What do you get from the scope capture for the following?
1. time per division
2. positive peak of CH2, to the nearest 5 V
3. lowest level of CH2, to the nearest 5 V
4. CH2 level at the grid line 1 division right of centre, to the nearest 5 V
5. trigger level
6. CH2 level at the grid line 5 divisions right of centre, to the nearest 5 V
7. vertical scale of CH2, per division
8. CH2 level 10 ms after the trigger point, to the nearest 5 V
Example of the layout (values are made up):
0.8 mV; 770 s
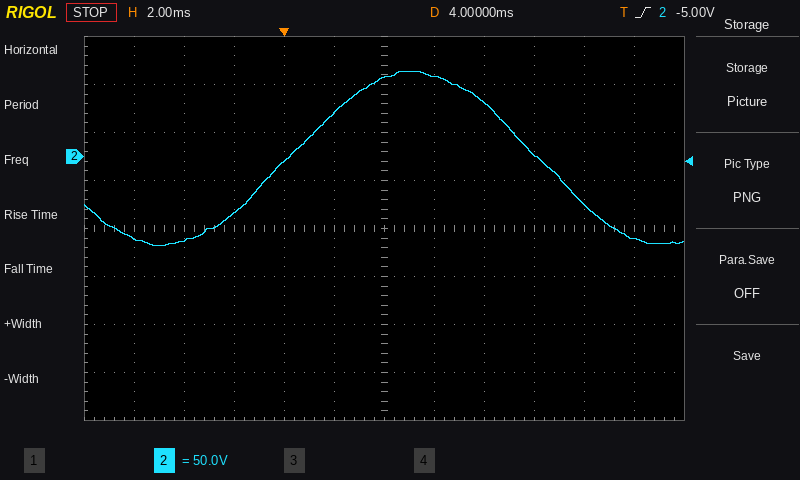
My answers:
2 ms; 90 V; -95 V; 85 V; -5.00 V; -85 V; 50 V; 0 V
